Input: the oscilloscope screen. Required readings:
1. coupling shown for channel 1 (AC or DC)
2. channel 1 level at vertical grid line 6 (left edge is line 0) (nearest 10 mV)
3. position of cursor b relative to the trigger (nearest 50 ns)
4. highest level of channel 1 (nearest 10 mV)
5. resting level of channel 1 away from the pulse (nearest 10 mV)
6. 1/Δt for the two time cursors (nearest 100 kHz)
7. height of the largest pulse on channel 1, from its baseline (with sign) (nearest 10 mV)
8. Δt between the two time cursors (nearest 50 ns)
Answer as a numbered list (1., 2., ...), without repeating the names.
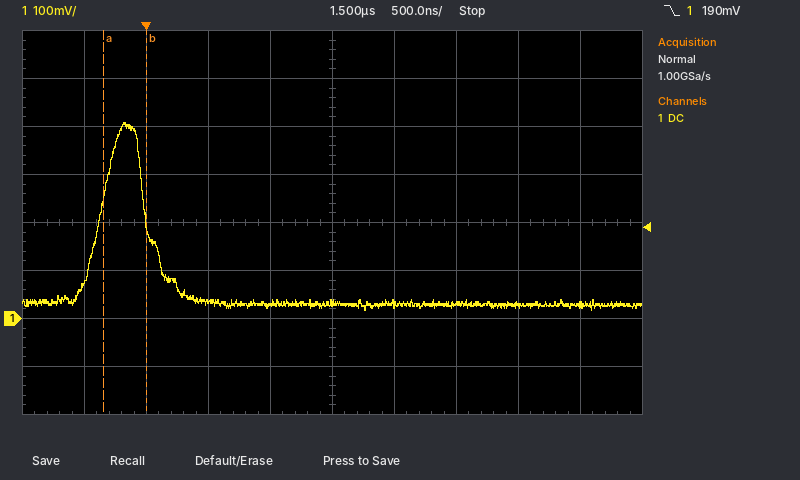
1. DC
2. 30 mV
3. 0 ns
4. 410 mV
5. 30 mV
6. 2.9 MHz
7. +380 mV
8. 350 ns
